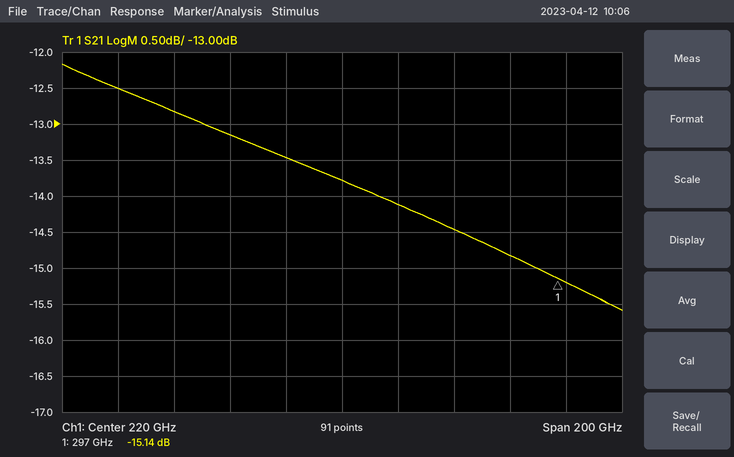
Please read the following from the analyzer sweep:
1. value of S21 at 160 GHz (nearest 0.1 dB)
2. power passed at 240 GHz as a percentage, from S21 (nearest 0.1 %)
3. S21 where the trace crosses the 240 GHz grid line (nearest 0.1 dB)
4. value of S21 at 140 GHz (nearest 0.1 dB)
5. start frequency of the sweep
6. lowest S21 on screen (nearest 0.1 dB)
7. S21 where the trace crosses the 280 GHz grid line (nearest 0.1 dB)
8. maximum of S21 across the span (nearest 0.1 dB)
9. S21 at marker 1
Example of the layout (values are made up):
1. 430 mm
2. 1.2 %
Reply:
1. -12.8 dB
2. 3.9 %
3. -14.1 dB
4. -12.5 dB
5. 120 GHz
6. -15.6 dB
7. -14.8 dB
8. -12.2 dB
9. -15.14 dB
